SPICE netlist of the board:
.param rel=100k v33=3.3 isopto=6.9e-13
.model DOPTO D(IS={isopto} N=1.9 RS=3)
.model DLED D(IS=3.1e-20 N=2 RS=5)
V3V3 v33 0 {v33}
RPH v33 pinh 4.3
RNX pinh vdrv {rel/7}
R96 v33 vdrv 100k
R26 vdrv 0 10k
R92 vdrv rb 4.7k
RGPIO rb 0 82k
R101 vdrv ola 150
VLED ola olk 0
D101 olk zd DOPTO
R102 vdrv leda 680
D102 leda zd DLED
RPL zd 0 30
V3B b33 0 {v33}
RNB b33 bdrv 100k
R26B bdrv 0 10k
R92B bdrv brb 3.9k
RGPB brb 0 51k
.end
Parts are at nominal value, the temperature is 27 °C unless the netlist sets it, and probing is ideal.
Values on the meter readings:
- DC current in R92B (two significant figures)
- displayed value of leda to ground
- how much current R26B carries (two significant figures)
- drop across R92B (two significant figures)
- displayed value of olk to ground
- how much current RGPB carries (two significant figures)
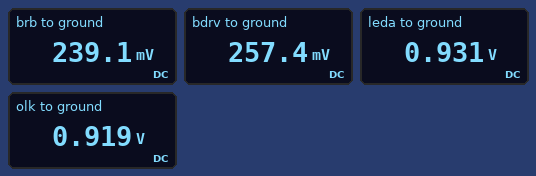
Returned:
4.7 µA
0.931 V
26 µA
18 mV
0.919 V
4.7 µA
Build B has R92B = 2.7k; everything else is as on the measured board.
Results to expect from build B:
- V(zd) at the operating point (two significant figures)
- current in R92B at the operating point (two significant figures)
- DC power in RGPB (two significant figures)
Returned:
2.6 mV
4.8 µA
1.2 µW
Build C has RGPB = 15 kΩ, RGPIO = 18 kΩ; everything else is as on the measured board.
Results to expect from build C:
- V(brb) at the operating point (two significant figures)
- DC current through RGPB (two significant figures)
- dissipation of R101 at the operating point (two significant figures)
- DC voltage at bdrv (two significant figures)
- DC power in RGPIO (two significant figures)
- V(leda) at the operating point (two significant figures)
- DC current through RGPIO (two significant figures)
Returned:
160 mV
11 µA
540 nW
200 mV
29 µW
910 mV
40 µA
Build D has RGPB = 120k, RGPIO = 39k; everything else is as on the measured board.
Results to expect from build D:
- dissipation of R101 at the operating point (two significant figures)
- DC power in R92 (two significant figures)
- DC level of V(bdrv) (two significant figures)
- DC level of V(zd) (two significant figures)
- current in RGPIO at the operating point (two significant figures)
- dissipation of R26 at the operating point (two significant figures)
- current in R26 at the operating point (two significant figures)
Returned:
880 nW
2.1 µW
280 mV
2.3 mV
21 µA
85 µW
92 µA
